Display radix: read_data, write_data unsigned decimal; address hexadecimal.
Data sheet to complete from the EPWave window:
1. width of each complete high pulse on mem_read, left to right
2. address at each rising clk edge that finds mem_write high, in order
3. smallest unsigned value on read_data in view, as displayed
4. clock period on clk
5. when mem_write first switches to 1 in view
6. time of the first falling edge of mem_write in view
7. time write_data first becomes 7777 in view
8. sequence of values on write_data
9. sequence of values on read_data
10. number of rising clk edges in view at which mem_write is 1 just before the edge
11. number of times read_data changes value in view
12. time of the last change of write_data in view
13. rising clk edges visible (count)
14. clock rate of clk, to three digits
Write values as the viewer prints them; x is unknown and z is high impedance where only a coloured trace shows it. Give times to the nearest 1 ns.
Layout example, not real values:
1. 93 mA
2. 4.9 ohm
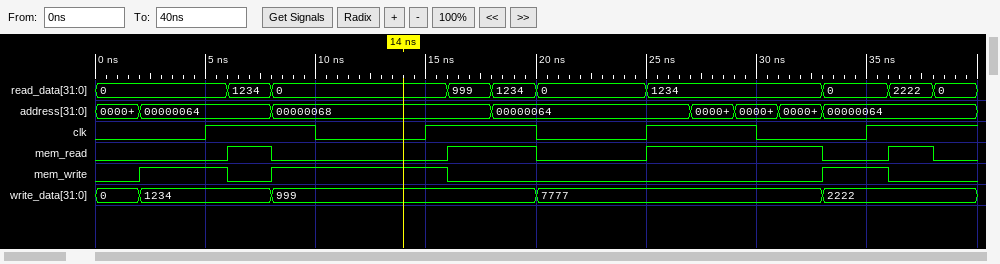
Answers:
1. 2 ns, 4 ns, 8 ns, 2 ns
2. 00000064, 00000068, 00000064
3. 0
4. 10 ns
5. 2 ns
6. 6 ns
7. 20 ns
8. 0, 1234, 999, 7777, 2222
9. 0, 1234, 0, 999, 1234, 0, 1234, 0, 2222, 0
10. 3
11. 9
12. 33 ns
13. 4
14. 100 MHz
